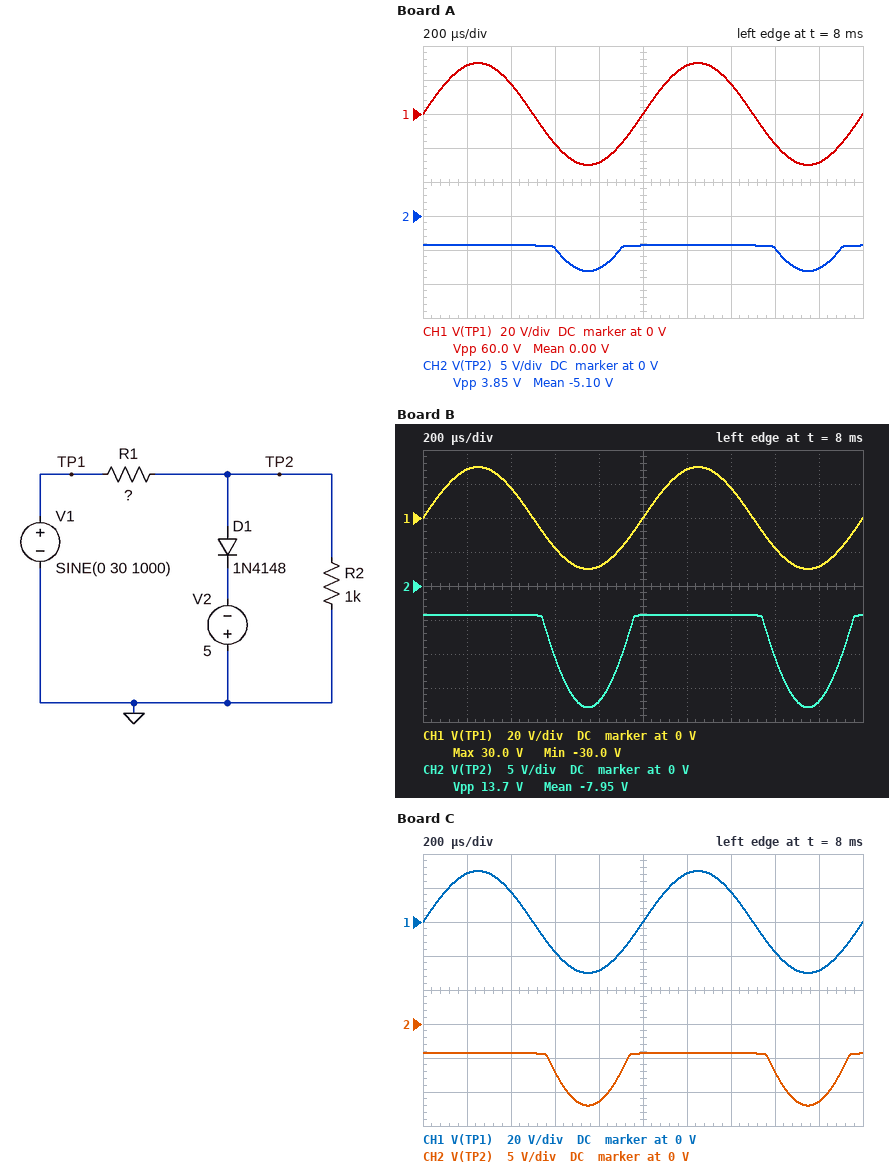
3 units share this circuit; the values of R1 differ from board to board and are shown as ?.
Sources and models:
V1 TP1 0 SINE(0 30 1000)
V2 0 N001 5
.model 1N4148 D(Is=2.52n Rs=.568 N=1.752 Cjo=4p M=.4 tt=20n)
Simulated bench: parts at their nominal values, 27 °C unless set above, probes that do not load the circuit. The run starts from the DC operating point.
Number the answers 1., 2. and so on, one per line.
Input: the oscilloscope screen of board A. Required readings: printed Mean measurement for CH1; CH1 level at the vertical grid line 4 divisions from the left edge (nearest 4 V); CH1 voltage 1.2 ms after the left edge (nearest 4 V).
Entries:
1. 0.00 V
2. -28 V
3. 28 V
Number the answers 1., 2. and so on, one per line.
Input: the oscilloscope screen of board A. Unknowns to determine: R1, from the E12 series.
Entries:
1. 2.7 kΩ
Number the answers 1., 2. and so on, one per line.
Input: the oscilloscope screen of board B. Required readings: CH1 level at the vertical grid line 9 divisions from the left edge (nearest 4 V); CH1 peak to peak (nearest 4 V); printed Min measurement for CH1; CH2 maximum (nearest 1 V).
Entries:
1. -28 V
2. 60 V
3. -30.0 V
4. -4 V
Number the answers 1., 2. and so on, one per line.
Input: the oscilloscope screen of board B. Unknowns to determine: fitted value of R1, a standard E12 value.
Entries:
1. 680 Ω
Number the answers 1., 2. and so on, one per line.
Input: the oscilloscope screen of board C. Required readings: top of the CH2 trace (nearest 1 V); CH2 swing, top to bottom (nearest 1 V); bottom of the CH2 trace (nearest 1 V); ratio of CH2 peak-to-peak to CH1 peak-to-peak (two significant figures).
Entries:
1. -4 V
2. 8 V
3. -12 V
4. 0.13
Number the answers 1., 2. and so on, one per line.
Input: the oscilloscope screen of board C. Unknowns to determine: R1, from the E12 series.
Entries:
1. 1.5 kΩ
